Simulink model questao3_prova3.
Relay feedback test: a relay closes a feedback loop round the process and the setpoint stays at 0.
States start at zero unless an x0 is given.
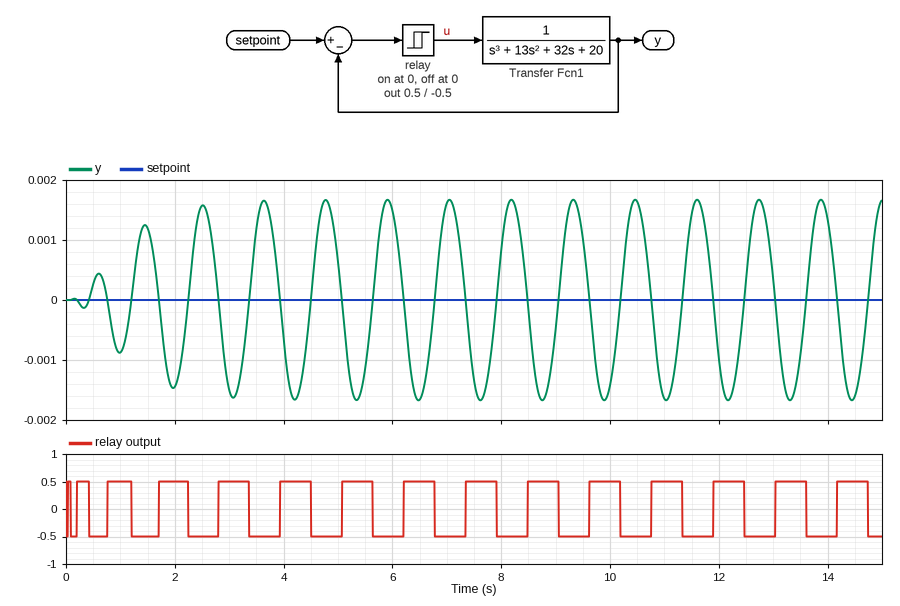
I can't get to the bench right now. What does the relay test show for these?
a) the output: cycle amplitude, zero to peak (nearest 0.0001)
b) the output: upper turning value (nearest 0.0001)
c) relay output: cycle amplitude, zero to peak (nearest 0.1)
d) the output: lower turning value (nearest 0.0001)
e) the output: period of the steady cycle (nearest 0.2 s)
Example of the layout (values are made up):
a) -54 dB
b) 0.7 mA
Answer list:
a) 0.0017
b) 0.0017
c) 0.5
d) -0.0017
e) 1.2 s
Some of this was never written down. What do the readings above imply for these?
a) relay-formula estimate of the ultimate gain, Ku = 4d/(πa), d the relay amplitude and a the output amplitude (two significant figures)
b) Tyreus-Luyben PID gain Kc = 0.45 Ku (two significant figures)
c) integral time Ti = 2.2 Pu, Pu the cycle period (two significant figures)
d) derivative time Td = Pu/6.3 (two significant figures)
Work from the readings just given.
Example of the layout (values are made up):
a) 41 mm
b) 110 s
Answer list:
a) 370
b) 170
c) 2.6 s
d) 0.19 s
